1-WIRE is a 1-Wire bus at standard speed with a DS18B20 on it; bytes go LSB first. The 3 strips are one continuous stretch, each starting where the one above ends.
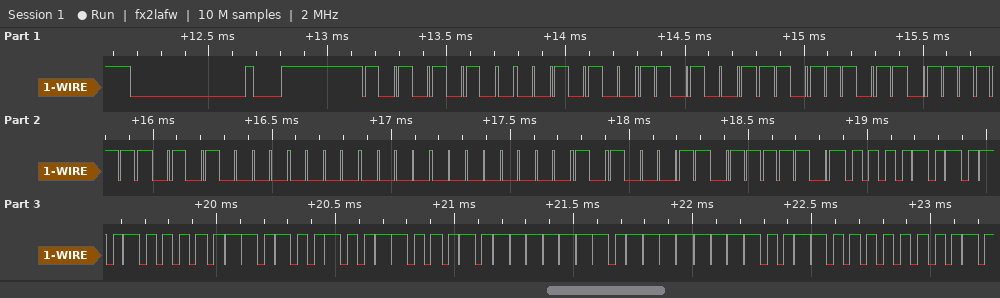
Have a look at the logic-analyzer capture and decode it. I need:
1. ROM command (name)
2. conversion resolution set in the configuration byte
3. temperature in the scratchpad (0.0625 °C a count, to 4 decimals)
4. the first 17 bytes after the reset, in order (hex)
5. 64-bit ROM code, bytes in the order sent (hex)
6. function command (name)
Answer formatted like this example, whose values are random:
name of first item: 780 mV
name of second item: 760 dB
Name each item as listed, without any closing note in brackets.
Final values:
ROM command: Match ROM
conversion resolution set in the configuration byte: 12 bits
temperature in the scratchpad: 85.0000 °C
the first 17 bytes after the reset, in order: 55 28 CB DD FE 0A 00 00 C5 BE 50 05 4B 46 7F FF 0C
64-bit ROM code, bytes in the order sent: 28 CB DD FE 0A 00 00 C5
function command: Read Scratchpad
